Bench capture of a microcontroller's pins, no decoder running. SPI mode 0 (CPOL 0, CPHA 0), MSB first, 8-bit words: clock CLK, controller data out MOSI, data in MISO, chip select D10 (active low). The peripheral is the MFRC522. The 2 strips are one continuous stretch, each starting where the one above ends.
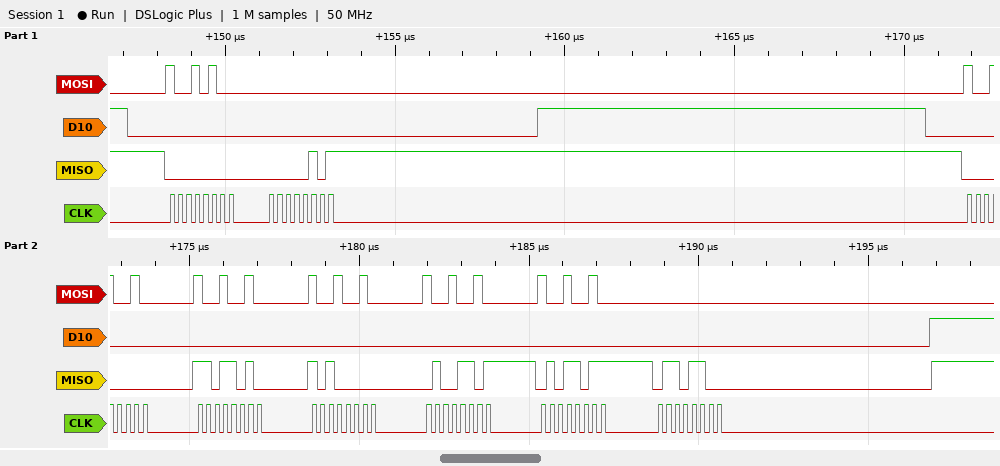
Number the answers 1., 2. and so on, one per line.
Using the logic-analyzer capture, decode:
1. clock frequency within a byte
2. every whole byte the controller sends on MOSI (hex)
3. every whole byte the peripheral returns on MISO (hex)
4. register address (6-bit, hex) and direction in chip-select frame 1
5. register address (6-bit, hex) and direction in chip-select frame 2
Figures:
1. 4 MHz
2. 0x94 0x00 0x92 0x92 0x92 0x92 0x92 0x00
3. 0x00 0x05 0x00 0xDA 0xA0 0x4D 0x5B 0x6C
4. 0x0A read
5. 0x09 read
